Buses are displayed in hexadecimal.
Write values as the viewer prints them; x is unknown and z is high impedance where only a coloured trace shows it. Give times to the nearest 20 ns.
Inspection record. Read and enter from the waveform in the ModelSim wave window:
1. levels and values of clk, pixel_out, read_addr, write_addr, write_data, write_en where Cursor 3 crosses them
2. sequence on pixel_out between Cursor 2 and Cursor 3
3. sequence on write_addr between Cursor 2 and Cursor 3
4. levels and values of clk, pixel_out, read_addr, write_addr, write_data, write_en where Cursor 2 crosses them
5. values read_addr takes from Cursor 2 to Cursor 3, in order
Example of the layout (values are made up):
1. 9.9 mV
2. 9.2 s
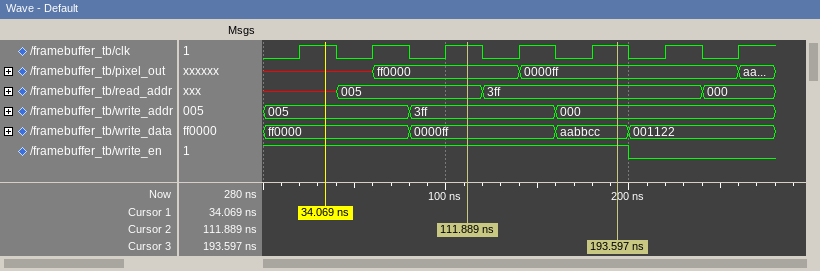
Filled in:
1. clk=1, pixel_out=0000ff, read_addr=3ff, write_addr=000, write_data=aabbcc, write_en=1
2. ff0000, 0000ff
3. 3ff, 000
4. clk=1, pixel_out=ff0000, read_addr=005, write_addr=3ff, write_data=0000ff, write_en=1
5. 005, 3ff
